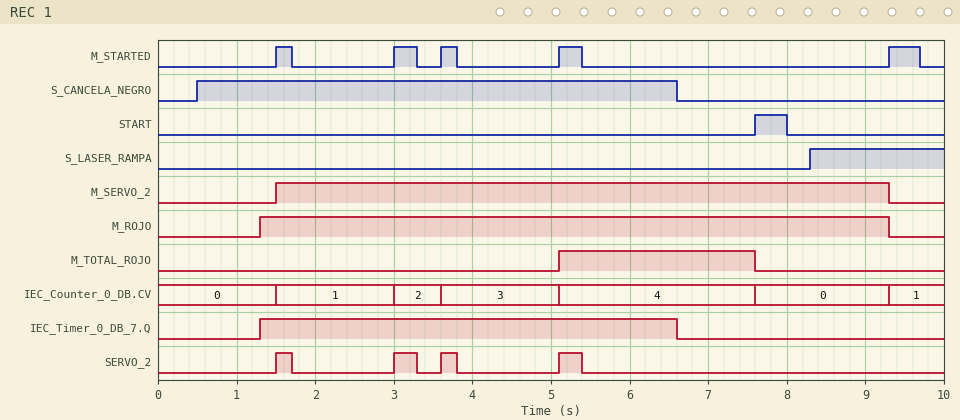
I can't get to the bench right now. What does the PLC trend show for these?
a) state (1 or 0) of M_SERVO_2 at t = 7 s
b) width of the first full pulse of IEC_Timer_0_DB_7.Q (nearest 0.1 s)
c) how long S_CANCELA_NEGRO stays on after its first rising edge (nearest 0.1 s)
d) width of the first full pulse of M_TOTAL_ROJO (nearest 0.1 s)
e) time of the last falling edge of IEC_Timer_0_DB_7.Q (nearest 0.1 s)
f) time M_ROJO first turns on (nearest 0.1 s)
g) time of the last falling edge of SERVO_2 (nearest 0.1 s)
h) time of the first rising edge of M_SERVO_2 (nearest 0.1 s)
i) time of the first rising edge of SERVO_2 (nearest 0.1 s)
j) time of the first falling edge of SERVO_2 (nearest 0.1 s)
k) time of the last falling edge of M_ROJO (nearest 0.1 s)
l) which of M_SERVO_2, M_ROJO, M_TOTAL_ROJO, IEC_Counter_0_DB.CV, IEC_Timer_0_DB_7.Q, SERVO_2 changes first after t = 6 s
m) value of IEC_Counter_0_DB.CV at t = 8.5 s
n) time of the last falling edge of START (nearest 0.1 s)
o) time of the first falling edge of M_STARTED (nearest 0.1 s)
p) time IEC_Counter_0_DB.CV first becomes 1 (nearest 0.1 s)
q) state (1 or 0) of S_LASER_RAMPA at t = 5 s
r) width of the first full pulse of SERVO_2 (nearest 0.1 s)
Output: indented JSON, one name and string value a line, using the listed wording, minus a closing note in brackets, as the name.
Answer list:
{
  "state (1 or 0) of M_SERVO_2 at t = 7 s": "1",
  "width of the first full pulse of IEC_Timer_0_DB_7.Q": "5.3 s",
  "how long S_CANCELA_NEGRO stays on after its first rising edge": "6.1 s",
  "width of the first full pulse of M_TOTAL_ROJO": "2.5 s",
  "time of the last falling edge of IEC_Timer_0_DB_7.Q": "6.6 s",
  "time M_ROJO first turns on": "1.3 s",
  "time of the last falling edge of SERVO_2": "5.4 s",
  "time of the first rising edge of M_SERVO_2": "1.5 s",
  "time of the first rising edge of SERVO_2": "1.5 s",
  "time of the first falling edge of SERVO_2": "1.7 s",
  "time of the last falling edge of M_ROJO": "9.3 s",
  "which of M_SERVO_2, M_ROJO, M_TOTAL_ROJO, IEC_Counter_0_DB.CV, IEC_Timer_0_DB_7.Q, SERVO_2 changes first after t = 6 s": "IEC_Timer_0_DB_7.Q",
  "value of IEC_Counter_0_DB.CV at t = 8.5 s": "0",
  "time of the last falling edge of START": "8.0 s",
  "time of the first falling edge of M_STARTED": "1.7 s",
  "time IEC_Counter_0_DB.CV first becomes 1": "1.5 s",
  "state (1 or 0) of S_LASER_RAMPA at t = 5 s": "0",
  "width of the first full pulse of SERVO_2": "0.2 s"
}
